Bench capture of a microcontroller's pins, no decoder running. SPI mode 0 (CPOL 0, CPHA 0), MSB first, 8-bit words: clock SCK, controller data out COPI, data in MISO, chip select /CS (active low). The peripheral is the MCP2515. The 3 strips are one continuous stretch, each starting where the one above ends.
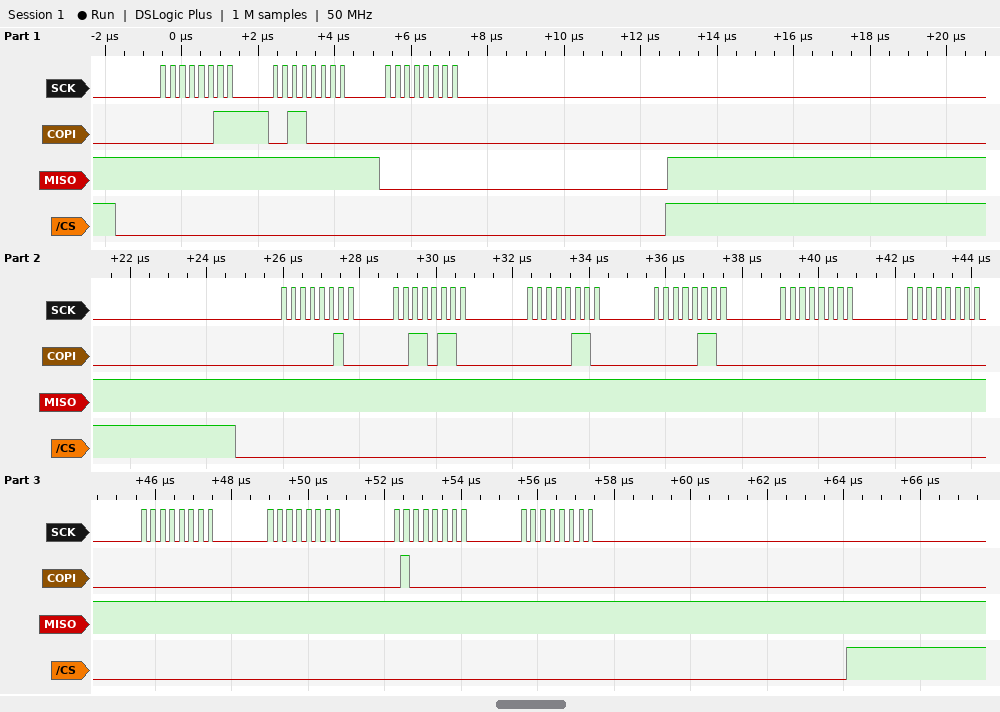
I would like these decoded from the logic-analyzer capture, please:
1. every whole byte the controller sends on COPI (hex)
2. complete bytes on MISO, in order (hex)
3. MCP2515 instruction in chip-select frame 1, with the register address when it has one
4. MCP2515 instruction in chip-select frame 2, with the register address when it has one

0x03 0x30 0x00 0x02 0x36 0x06 0x06 0x00 0x00 0x00 0x00 0x40 0x00
0xFF 0xFF 0x00 0xFF 0xFF 0xFF 0xFF 0xFF 0xFF 0xFF 0xFF 0xFF 0xFF
READ 0x30
WRITE 0x36
